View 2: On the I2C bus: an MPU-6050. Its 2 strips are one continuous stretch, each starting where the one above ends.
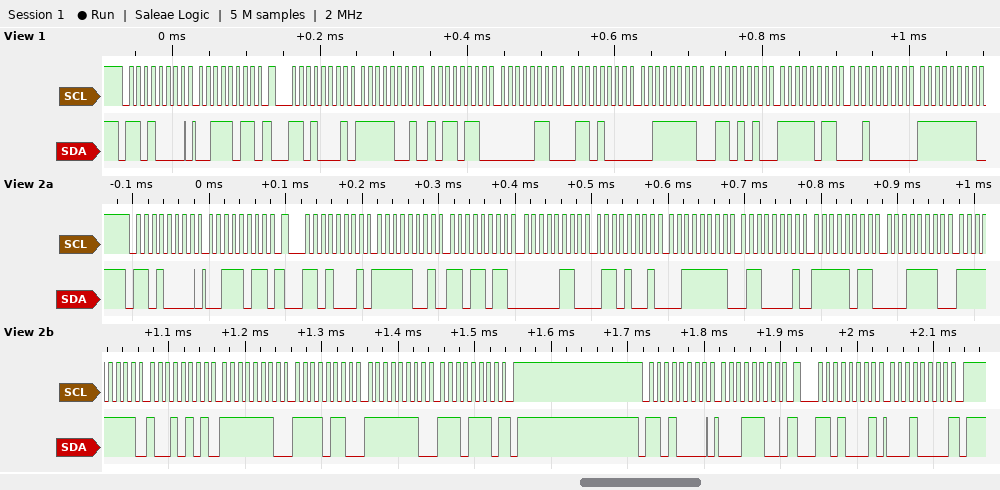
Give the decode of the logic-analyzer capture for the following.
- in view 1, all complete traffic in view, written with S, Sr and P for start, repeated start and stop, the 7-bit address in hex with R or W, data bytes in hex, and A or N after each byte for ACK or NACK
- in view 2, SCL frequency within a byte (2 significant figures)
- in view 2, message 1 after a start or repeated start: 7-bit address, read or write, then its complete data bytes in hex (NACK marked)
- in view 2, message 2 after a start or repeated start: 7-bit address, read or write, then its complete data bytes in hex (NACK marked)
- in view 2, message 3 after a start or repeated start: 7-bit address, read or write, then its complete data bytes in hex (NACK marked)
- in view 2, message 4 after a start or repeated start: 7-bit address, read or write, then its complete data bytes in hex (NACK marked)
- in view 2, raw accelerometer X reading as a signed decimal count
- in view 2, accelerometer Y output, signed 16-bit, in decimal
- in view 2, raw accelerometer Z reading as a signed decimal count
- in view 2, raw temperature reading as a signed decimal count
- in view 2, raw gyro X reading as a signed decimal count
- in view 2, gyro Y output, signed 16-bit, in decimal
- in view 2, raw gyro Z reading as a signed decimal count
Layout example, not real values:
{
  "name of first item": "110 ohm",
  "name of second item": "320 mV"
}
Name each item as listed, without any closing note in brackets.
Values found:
{
  "in view 1, all complete traffic in view, written with S, Sr and P for start, repeated start and stop, the 7-bit address in hex with R or W, data bytes in hex, and A or N after each byte for ACK or NACK": "S 68W A 3B A Sr 68R A F9 A B6 A 06 A 68 A 3F A 6A A FB A 20 A FF A",
  "in view 2, SCL frequency within a byte": "100 kHz",
  "in view 2, message 1 after a start or repeated start: 7-bit address, read or write, then its complete data bytes in hex": "0x68 write: 3B",
  "in view 2, message 2 after a start or repeated start: 7-bit address, read or write, then its complete data bytes in hex": "0x68 read: F9 DB 06 69 3F 61 FB 1E FF 95 FE F6 FE EE NACK",
  "in view 2, message 3 after a start or repeated start: 7-bit address, read or write, then its complete data bytes in hex": "0x68 write: 1C",
  "in view 2, message 4 after a start or repeated start: 7-bit address, read or write, then its complete data bytes in hex": "0x68 read: 10 NACK",
  "in view 2, raw accelerometer X reading as a signed decimal count": "-1573",
  "in view 2, accelerometer Y output, signed 16-bit, in decimal": "1641",
  "in view 2, raw accelerometer Z reading as a signed decimal count": "16225",
  "in view 2, raw temperature reading as a signed decimal count": "-1250",
  "in view 2, raw gyro X reading as a signed decimal count": "-107",
  "in view 2, gyro Y output, signed 16-bit, in decimal": "-266",
  "in view 2, raw gyro Z reading as a signed decimal count": "-274"
}
